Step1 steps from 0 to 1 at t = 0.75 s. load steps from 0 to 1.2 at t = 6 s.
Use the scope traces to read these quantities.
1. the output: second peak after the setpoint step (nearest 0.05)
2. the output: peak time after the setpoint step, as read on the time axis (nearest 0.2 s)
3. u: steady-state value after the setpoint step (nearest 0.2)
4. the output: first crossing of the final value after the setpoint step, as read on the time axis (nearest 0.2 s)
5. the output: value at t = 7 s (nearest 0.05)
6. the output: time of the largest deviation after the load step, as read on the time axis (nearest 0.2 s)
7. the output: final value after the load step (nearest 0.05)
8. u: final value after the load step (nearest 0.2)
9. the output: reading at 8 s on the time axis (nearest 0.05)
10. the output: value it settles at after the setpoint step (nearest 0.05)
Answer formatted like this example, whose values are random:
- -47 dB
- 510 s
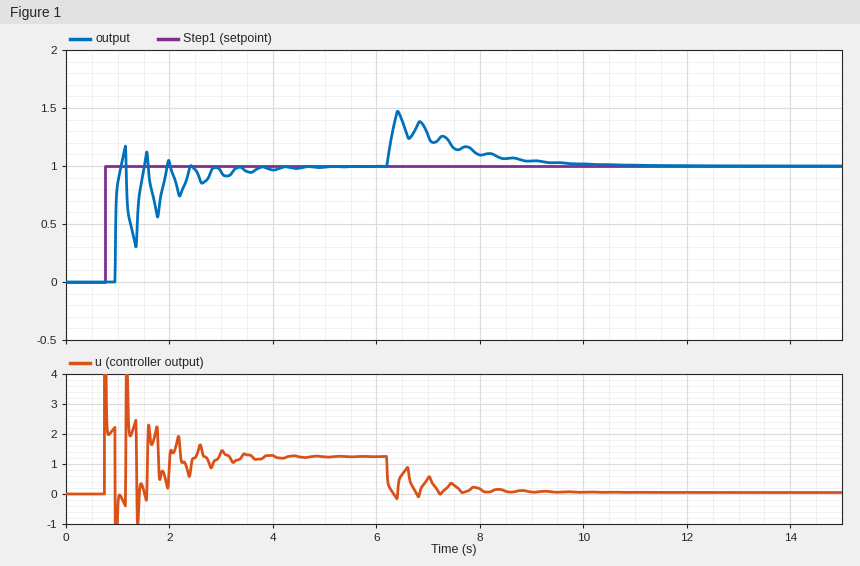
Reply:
- 1.10
- 1.2 s
- 1.2
- 1.0 s
- 1.25
- 6.4 s
- 1.00
- 0.0
- 1.10
- 1.00
